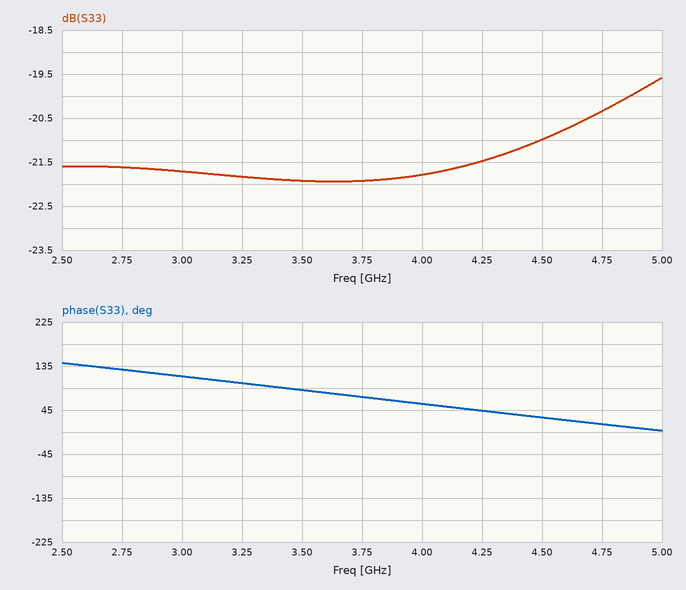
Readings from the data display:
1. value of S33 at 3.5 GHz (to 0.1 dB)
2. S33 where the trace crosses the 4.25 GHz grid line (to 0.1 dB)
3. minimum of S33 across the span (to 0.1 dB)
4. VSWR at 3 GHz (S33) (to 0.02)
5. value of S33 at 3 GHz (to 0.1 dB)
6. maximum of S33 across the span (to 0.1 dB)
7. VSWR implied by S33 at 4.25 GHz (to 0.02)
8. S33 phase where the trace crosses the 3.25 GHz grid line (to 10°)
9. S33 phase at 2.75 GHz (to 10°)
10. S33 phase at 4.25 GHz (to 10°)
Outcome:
-21.9 dB
-21.5 dB
-21.9 dB
1.18
-21.7 dB
-19.6 dB
1.18
100°
130°
40°
